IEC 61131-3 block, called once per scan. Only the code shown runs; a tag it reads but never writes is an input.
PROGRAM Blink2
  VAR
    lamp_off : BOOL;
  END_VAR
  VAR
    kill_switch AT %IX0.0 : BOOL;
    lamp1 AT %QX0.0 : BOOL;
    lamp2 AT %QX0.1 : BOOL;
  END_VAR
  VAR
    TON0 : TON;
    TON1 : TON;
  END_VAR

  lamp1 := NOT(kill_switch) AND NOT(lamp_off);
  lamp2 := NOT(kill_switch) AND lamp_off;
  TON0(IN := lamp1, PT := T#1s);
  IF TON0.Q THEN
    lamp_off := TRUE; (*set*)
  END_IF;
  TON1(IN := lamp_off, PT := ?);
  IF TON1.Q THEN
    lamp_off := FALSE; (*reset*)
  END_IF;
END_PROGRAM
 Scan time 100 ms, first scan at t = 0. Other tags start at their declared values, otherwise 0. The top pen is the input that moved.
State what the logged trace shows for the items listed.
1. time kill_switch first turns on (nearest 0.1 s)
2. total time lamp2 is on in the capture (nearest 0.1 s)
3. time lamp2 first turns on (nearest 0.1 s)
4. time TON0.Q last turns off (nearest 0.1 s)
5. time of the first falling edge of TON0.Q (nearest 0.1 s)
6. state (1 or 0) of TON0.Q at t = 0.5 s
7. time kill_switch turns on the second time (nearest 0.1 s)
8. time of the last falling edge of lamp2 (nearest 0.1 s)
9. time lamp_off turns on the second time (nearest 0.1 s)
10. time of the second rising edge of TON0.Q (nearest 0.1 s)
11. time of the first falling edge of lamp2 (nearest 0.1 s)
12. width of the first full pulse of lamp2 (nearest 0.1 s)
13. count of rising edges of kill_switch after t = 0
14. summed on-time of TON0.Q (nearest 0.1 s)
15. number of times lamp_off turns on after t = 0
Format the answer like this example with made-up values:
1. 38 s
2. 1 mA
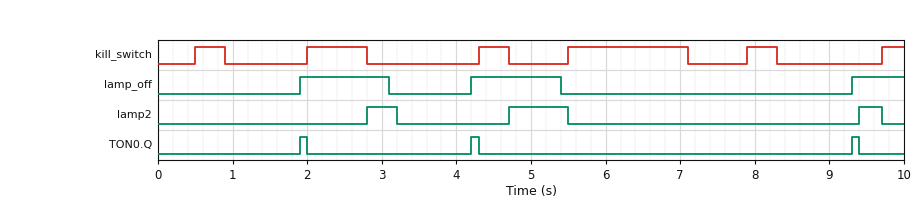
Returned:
1. 0.5 s
2. 1.5 s
3. 2.8 s
4. 9.4 s
5. 2.0 s
6. 0
7. 2.0 s
8. 9.7 s
9. 4.2 s
10. 4.2 s
11. 3.2 s
12. 0.4 s
13. 6
14. 0.3 s
15. 3
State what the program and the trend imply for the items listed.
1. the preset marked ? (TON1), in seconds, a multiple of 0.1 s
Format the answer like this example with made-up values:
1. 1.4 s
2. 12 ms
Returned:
1. 1.2 s
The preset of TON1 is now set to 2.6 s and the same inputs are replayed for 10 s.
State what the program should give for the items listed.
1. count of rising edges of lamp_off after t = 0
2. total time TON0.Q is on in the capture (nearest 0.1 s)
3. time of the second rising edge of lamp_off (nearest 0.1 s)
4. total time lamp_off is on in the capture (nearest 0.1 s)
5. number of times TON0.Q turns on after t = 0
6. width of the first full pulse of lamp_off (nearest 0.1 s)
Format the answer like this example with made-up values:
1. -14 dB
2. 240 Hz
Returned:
1. 2
2. 0.2 s
3. 9.3 s
4. 3.3 s
5. 2
6. 2.6 s
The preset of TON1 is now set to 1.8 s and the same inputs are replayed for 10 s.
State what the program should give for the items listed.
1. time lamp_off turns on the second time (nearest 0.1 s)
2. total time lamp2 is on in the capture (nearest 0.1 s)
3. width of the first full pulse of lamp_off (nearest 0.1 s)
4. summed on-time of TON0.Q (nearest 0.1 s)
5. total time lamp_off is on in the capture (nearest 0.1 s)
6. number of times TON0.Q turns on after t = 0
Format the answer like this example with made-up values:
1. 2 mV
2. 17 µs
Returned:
1. 9.3 s
2. 1.3 s
3. 1.8 s
4. 0.2 s
5. 2.5 s
6. 2
